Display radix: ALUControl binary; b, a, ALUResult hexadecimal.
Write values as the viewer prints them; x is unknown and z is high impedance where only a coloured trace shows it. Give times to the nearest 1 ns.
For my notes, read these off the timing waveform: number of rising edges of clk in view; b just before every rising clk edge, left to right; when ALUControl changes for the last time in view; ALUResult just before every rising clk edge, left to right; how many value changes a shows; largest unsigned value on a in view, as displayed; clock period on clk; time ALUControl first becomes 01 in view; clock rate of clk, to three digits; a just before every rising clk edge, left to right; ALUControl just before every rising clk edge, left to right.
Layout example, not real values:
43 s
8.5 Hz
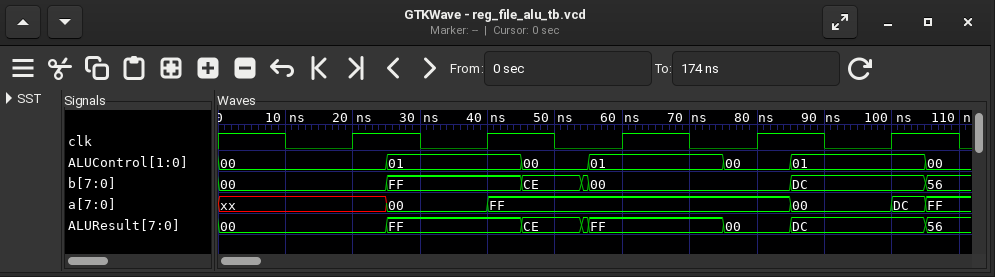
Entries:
5
00, FF, 00, 00, DC
105 ns
00, FF, FF, 00, DC
5
FF
20 ns
25 ns
50.0 MHz
xx, 00, FF, FF, 00
00, 01, 01, 00, 01
